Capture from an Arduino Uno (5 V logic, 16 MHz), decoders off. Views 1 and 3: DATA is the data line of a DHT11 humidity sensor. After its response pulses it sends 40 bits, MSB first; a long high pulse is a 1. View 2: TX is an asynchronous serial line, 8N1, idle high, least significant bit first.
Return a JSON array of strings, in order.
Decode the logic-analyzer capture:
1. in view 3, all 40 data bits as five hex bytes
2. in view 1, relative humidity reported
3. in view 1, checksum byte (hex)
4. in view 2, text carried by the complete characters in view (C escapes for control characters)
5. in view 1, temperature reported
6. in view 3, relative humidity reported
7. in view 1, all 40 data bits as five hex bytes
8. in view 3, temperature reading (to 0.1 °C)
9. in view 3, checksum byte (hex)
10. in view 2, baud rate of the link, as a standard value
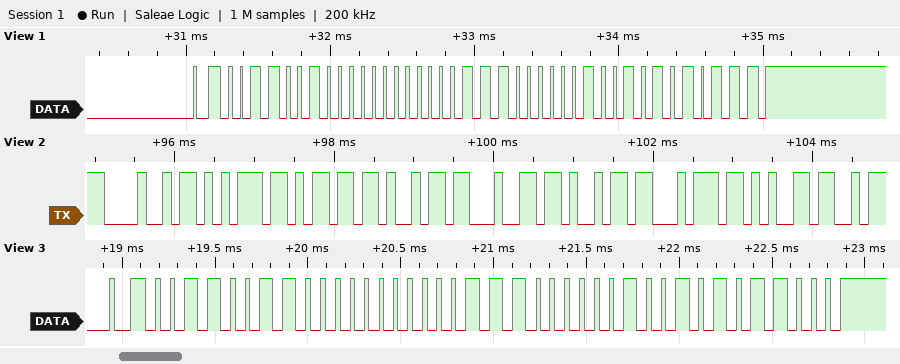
["33 00 1C 09 58", "50 %", "0x57", "\"Humidite\"", "28.9 °C", "51 %", "32 00 1C 09 57", "28.9 °C", "0x58", "9600 baud"]
